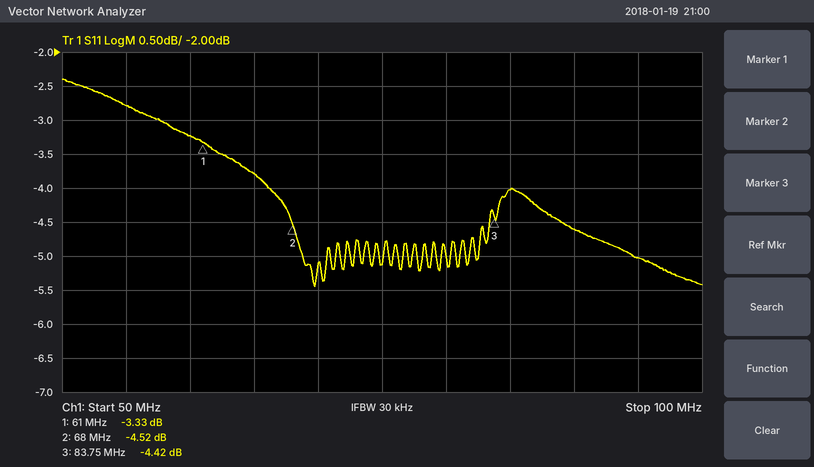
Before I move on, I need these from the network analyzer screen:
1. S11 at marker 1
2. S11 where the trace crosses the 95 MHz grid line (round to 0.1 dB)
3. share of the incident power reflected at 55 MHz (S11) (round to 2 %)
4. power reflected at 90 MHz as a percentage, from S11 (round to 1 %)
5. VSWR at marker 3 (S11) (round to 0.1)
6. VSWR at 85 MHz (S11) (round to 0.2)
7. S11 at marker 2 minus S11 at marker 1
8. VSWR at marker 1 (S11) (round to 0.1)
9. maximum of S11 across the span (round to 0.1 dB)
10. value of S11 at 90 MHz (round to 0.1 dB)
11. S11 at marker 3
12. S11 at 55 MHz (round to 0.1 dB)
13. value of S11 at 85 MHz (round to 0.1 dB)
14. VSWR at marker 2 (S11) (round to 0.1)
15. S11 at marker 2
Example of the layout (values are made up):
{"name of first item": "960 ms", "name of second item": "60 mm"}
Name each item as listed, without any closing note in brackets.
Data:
{"S11 at marker 1": "-3.33 dB", "S11 where the trace crosses the 95 MHz grid line": "-5.0 dB", "share of the incident power reflected at 55 MHz (S11)": "52 %", "power reflected at 90 MHz as a percentage, from S11": "35 %", "VSWR at marker 3 (S11)": "4.0", "VSWR at 85 MHz (S11)": "4.4", "S11 at marker 2 minus S11 at marker 1": "-1.19 dB", "VSWR at marker 1 (S11)": "5.3", "maximum of S11 across the span": "-2.4 dB", "value of S11 at 90 MHz": "-4.6 dB", "S11 at marker 3": "-4.42 dB", "S11 at 55 MHz": "-2.8 dB", "value of S11 at 85 MHz": "-4.0 dB", "VSWR at marker 2 (S11)": "3.9", "S11 at marker 2": "-4.52 dB"}
